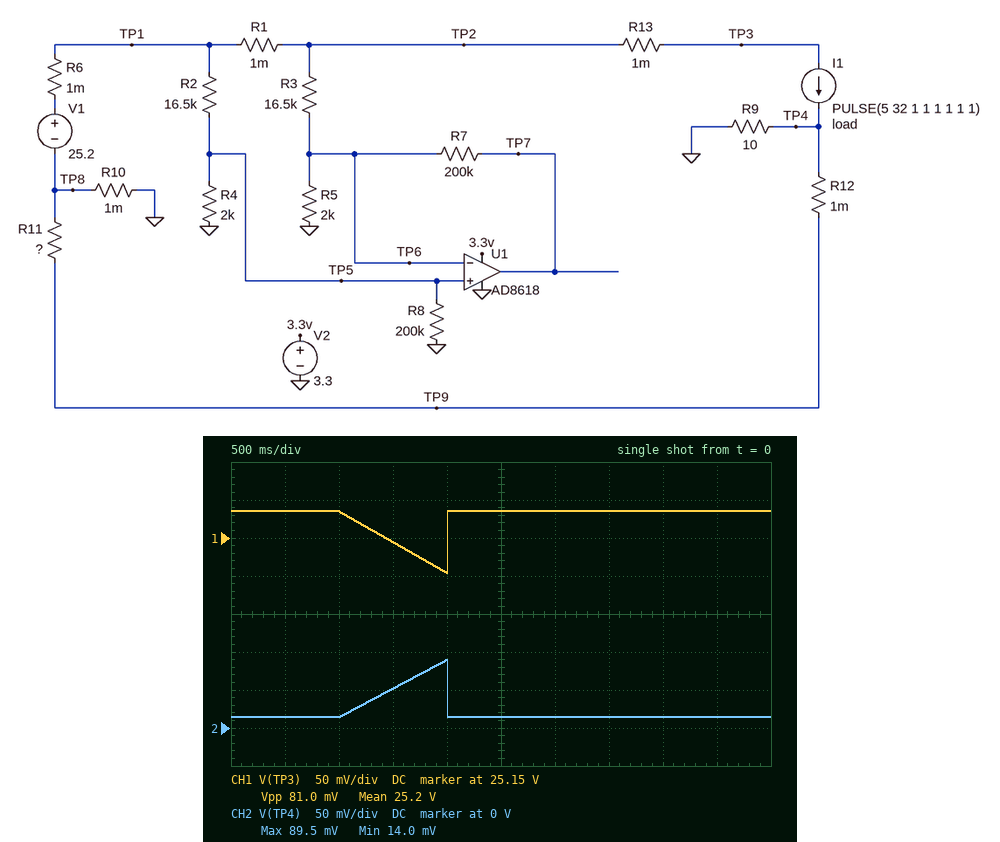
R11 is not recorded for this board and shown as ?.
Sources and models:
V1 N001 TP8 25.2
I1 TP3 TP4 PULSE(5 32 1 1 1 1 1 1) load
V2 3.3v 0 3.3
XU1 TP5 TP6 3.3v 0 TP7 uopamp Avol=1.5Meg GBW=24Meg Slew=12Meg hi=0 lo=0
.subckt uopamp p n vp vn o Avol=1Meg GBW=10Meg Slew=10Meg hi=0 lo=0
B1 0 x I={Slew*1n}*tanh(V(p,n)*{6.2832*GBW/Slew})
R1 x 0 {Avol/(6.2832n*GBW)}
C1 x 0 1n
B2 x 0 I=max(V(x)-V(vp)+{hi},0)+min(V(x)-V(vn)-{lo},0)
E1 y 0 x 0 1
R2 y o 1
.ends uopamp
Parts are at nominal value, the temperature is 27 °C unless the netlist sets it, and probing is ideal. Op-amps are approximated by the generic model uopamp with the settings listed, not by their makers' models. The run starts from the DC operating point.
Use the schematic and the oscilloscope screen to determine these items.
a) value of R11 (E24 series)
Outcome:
1.8 mΩ
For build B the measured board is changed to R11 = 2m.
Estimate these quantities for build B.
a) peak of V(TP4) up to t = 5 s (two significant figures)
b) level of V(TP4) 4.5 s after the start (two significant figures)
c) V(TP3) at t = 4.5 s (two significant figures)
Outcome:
96 mV
15 mV
25 V
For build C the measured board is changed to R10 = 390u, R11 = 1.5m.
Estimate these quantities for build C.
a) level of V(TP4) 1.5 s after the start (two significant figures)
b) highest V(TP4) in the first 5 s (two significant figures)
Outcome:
46 mV
80 mV
